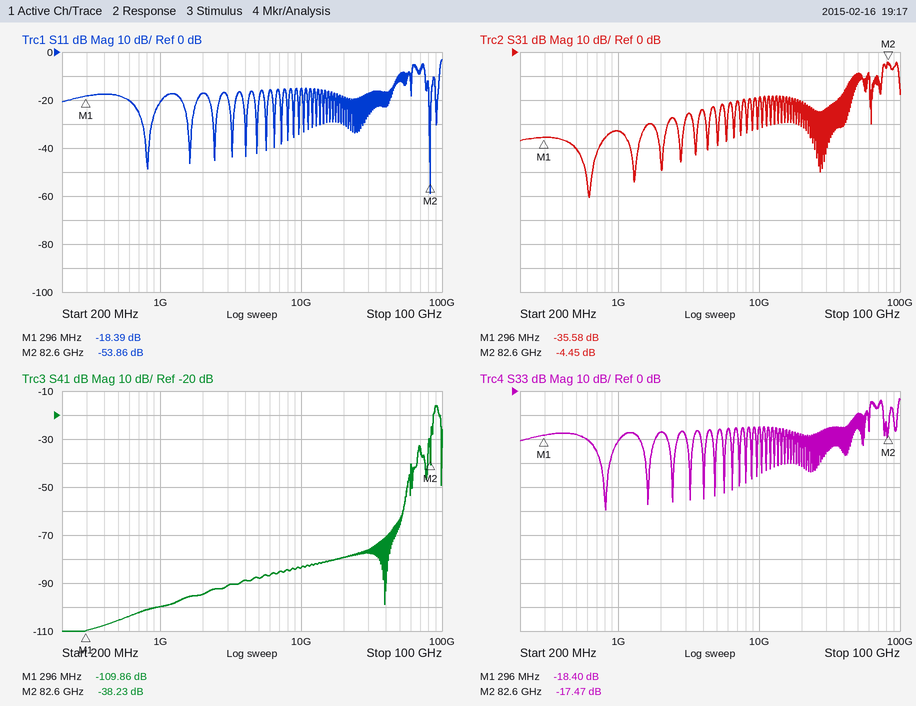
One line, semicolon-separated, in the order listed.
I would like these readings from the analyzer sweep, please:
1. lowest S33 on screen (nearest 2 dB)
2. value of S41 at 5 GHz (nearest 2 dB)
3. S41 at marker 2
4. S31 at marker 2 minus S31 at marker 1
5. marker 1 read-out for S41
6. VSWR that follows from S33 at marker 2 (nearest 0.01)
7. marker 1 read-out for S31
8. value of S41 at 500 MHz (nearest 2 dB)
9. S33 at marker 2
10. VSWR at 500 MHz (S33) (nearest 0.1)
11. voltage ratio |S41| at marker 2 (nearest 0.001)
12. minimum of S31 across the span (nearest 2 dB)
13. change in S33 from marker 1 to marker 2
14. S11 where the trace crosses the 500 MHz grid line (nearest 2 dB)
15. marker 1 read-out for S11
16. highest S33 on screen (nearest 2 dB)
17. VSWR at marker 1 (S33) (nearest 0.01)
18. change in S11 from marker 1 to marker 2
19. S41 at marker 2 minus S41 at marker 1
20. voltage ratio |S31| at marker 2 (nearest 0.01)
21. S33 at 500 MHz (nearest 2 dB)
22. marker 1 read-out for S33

-50 dB; -88 dB; -38.23 dB; 31.13 dB; -109.86 dB; 1.31; -35.58 dB; -106 dB; -17.47 dB; 1.3; 0.012; -60 dB; 0.93 dB; -18 dB; -18.39 dB; -4 dB; 1.27; -35.47 dB; 71.63 dB; 0.60; -18 dB; -18.40 dB
